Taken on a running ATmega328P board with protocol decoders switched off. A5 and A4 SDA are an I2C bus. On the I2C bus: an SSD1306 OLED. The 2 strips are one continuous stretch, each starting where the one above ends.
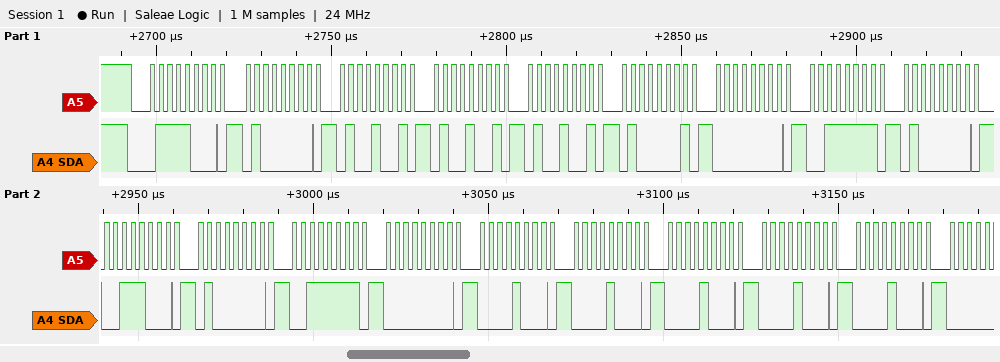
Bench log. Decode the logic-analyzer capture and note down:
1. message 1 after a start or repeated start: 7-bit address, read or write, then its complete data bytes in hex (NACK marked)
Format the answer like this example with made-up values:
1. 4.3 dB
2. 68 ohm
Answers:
1. 0x3C write: 40 49 49 49 41 00 3F 40 38 40 3F 00 08 08 08 08 08
